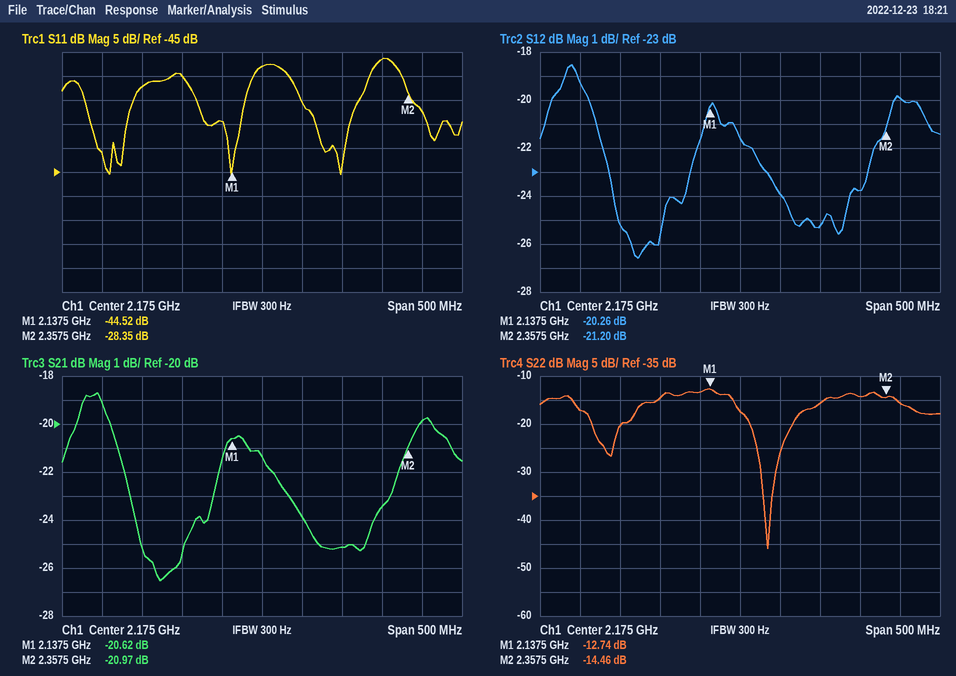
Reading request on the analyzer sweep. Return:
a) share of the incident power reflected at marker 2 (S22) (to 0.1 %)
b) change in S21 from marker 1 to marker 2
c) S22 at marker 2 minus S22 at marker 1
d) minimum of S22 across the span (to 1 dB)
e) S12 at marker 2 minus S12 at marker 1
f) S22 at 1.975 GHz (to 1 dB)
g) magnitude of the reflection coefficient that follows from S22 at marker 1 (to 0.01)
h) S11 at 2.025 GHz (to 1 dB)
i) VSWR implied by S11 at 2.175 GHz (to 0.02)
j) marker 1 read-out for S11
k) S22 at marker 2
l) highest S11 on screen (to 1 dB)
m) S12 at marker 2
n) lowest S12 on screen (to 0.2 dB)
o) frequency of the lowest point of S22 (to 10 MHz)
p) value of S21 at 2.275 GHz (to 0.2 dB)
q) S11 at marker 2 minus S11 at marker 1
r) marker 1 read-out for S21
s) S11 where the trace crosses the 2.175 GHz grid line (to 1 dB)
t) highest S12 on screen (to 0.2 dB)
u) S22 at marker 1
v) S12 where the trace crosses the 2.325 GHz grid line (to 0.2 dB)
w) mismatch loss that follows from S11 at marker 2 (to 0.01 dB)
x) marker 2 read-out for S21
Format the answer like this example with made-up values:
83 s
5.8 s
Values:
3.6 %
-0.35 dB
-1.72 dB
-46 dB
-0.94 dB
-17 dB
0.23
-27 dB
1.16
-44.52 dB
-14.46 dB
-21 dB
-21.20 dB
-26.6 dB
2.21 GHz
-25.2 dB
16.17 dB
-20.62 dB
-23 dB
-18.6 dB
-12.74 dB
-23.8 dB
0.01 dB
-20.97 dB
